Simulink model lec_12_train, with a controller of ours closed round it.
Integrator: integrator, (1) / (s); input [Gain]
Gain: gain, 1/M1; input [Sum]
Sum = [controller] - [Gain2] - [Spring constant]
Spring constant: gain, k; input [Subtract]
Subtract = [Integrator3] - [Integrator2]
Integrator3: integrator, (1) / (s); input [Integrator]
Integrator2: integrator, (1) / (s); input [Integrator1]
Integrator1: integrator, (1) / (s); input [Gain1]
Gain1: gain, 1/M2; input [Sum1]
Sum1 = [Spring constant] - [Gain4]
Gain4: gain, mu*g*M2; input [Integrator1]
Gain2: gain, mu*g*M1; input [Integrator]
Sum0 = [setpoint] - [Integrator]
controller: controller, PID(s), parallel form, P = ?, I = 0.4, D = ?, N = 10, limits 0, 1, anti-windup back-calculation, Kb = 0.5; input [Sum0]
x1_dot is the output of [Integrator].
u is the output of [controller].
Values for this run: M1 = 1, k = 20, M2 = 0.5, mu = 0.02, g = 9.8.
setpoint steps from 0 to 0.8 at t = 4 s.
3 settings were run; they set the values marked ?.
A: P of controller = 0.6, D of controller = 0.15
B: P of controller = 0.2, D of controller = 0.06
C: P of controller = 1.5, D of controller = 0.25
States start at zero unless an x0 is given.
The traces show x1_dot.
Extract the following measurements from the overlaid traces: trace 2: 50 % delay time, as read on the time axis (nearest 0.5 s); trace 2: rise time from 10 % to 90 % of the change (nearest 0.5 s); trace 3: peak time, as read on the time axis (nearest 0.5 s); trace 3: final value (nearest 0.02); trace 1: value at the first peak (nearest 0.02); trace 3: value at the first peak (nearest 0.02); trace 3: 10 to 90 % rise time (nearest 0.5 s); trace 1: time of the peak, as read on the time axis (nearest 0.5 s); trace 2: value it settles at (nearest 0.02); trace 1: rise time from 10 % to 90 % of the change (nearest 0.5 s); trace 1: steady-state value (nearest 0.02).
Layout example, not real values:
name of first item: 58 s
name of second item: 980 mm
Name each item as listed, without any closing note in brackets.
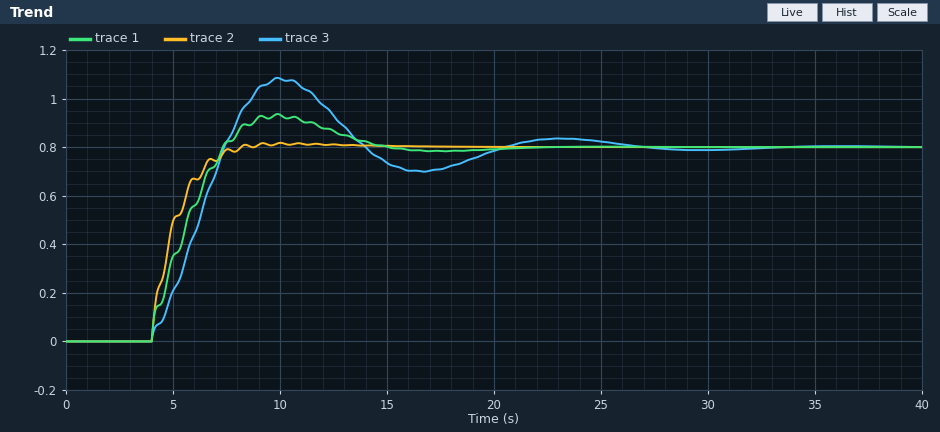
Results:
trace 2: 50 % delay time, as read on the time axis: 5.0 s
trace 2: rise time from 10 % to 90 % of the change: 2.5 s
trace 3: peak time, as read on the time axis: 10.0 s
trace 3: final value: 0.80
trace 1: value at the first peak: 0.94
trace 3: value at the first peak: 1.08
trace 3: 10 to 90 % rise time: 2.5 s
trace 1: time of the peak, as read on the time axis: 10.0 s
trace 2: value it settles at: 0.80
trace 1: rise time from 10 % to 90 % of the change: 3.0 s
trace 1: steady-state value: 0.80
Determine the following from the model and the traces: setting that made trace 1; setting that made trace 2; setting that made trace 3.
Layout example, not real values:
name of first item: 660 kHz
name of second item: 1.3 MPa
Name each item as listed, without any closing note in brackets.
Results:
setting that made trace 1: A
setting that made trace 2: C
setting that made trace 3: B
